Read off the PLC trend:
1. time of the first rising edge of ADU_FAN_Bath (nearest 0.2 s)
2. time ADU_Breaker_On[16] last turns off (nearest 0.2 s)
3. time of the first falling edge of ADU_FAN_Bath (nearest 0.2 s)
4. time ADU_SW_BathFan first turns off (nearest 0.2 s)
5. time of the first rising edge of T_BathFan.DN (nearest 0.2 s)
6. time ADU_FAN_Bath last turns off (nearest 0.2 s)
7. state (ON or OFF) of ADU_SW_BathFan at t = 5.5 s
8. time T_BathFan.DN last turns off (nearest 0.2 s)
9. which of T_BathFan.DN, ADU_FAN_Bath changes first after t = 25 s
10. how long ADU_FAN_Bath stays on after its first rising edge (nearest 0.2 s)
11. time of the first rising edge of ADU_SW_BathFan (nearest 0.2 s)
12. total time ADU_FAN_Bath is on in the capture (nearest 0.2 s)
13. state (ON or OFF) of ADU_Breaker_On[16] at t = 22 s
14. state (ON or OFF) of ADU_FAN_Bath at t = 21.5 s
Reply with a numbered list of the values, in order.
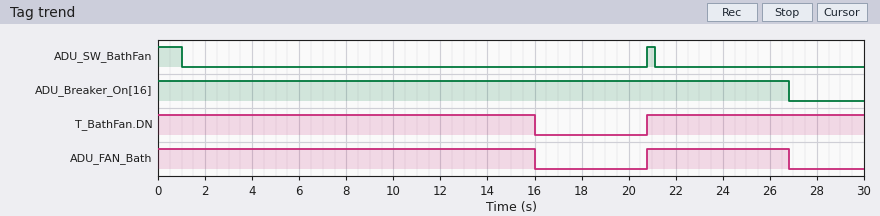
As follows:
1. 20.8 s
2. 26.8 s
3. 16.0 s
4. 1.0 s
5. 20.8 s
6. 26.8 s
7. OFF
8. 16.0 s
9. ADU_FAN_Bath
10. 6.0 s
11. 20.8 s
12. 22.0 s
13. ON
14. ON
